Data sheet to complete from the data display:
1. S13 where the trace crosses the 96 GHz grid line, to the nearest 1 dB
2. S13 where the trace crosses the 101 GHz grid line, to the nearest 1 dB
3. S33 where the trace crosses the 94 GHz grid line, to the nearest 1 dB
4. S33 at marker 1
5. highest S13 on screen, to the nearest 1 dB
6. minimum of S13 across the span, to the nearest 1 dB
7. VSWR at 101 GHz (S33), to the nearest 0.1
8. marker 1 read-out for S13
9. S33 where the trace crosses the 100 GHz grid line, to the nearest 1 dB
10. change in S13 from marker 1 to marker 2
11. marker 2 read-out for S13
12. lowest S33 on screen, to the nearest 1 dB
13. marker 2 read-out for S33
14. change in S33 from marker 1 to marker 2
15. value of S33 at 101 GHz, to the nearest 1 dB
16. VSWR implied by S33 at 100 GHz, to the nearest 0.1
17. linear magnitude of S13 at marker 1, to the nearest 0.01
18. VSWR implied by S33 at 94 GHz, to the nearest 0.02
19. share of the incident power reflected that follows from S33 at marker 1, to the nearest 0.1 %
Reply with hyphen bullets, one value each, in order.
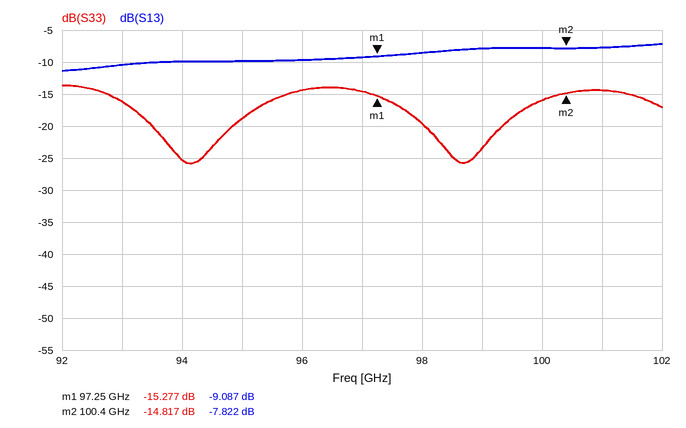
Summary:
- -10 dB
- -8 dB
- -25 dB
- -15.277 dB
- -7 dB
- -11 dB
- 1.5
- -9.087 dB
- -16 dB
- 1.265 dB
- -7.822 dB
- -26 dB
- -14.817 dB
- 0.460 dB
- -14 dB
- 1.4
- 0.35
- 1.12
- 3.0 %
